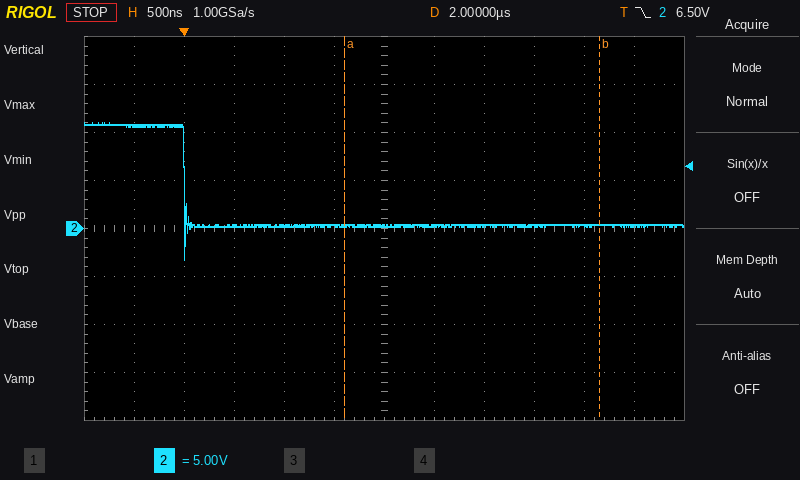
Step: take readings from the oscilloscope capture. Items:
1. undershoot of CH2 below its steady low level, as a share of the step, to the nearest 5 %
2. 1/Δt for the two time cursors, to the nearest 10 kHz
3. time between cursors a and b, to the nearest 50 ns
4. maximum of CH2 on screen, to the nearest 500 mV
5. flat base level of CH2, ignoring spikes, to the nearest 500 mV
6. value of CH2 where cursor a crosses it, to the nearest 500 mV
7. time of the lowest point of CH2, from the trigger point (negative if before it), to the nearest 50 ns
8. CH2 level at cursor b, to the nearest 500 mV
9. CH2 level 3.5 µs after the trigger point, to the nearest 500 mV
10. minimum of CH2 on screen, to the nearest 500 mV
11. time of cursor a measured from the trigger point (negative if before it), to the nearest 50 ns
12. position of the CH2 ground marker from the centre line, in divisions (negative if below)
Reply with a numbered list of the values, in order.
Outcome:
1. 35 %
2. 390 kHz
3. 2.55 µs
4. 11.0 V
5. 500 mV
6. 500 mV
7. 0 ns
8. 500 mV
9. 500 mV
10. -3.0 V
11. +1.60 µs
12. 0.0 div
